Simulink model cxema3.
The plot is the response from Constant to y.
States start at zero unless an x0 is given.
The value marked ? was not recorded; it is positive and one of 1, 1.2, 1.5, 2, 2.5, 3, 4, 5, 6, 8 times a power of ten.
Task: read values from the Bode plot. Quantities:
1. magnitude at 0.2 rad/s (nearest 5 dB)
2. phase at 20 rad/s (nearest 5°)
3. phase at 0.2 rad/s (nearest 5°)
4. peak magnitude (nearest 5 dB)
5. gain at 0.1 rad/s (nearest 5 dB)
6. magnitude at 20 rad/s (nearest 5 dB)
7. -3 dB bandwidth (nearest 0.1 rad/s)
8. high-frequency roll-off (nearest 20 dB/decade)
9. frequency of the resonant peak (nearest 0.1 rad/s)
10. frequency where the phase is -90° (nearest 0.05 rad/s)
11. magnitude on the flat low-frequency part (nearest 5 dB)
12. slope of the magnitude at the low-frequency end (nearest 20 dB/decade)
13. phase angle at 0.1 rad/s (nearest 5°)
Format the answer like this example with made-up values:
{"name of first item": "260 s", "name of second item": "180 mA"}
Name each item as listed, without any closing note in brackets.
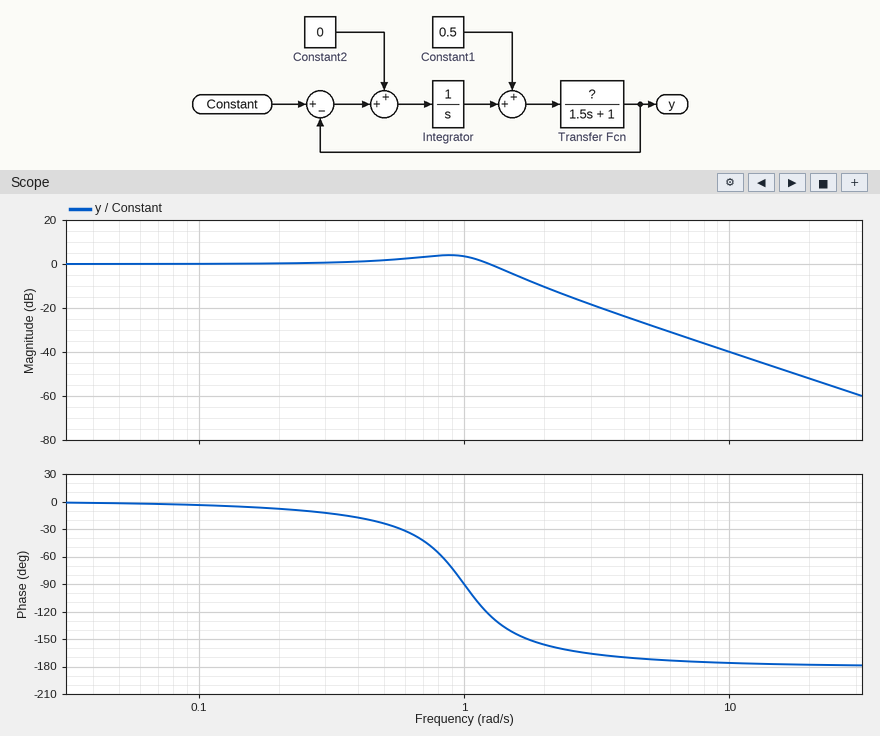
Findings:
{"magnitude at 0.2 rad/s": "0 dB", "phase at 20 rad/s": "-180°", "phase at 0.2 rad/s": "-10°", "peak magnitude": "5 dB", "gain at 0.1 rad/s": "0 dB", "magnitude at 20 rad/s": "-50 dB", "-3 dB bandwidth": "1.4 rad/s", "high-frequency roll-off": "-40 dB/decade", "frequency of the resonant peak": "0.9 rad/s", "frequency where the phase is -90°": "1.00 rad/s", "magnitude on the flat low-frequency part": "0 dB", "slope of the magnitude at the low-frequency end": "0 dB/decade", "phase angle at 0.1 rad/s": "-5°"}
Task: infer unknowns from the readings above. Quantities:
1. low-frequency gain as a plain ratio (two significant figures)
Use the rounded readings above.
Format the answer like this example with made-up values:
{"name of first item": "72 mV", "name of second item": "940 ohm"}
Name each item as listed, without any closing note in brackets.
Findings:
{"low-frequency gain as a plain ratio": "1.0"}
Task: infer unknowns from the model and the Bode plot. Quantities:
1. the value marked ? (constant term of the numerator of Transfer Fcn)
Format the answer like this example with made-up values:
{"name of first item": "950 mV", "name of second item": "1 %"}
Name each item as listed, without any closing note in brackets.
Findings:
{"the value marked ?": "1.5"}
